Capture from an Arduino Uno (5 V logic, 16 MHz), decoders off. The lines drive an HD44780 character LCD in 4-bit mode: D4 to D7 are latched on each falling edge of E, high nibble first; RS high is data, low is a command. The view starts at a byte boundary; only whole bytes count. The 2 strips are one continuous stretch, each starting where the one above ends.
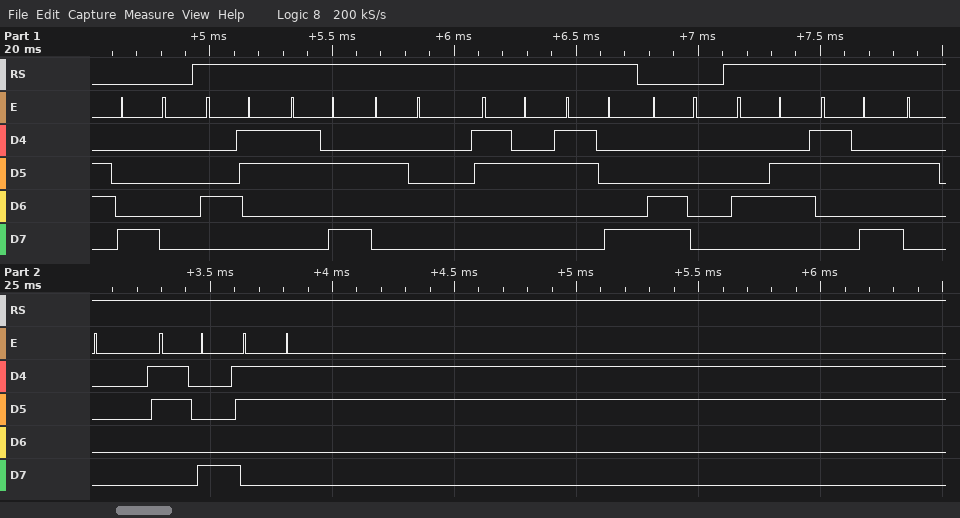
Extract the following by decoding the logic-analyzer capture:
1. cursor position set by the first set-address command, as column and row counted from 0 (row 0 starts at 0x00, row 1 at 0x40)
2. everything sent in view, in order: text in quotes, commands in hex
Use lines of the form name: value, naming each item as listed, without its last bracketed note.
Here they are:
cursor position set by the first set-address command, as column and row counted from 0: column 0, row 0
everything sent in view, in order: text in quotes, commands in hex: 0x80 "C: 28" 0xC0 "F: 83"
